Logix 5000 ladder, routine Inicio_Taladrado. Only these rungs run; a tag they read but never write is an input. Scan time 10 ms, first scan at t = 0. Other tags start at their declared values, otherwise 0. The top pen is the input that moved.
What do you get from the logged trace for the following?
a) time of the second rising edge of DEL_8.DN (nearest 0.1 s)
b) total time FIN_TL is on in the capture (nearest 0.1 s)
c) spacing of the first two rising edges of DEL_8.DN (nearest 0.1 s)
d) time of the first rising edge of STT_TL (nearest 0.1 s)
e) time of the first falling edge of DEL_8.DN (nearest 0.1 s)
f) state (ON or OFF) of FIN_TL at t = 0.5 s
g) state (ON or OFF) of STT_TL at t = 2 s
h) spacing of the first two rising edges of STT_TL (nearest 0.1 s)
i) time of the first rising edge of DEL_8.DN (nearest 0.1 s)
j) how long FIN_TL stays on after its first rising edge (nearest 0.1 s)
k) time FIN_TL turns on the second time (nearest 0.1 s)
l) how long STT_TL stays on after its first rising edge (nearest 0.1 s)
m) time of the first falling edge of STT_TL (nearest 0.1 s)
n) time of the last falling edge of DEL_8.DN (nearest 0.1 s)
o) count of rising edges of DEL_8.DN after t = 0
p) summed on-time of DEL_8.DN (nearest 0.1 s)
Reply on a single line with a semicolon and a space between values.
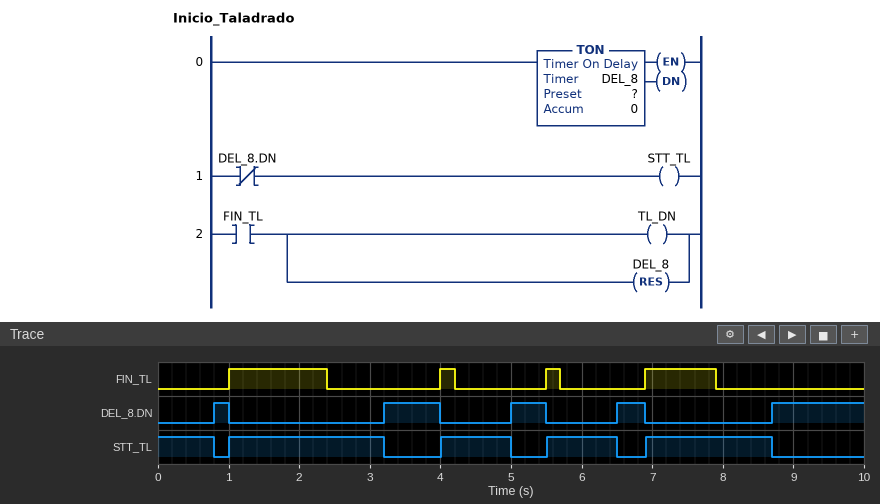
3.2 s; 2.8 s; 2.4 s; 1.0 s; 1.0 s; OFF; ON; 3.0 s; 0.8 s; 1.4 s; 4.0 s; 2.2 s; 0.8 s; 6.9 s; 5; 3.2 s
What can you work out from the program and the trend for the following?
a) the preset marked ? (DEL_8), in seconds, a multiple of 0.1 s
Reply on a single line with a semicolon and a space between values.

0.8 s
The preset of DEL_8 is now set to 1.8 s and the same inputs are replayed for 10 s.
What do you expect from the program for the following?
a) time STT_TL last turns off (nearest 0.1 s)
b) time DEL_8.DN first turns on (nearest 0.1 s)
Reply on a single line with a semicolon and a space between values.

9.7 s; 9.7 s
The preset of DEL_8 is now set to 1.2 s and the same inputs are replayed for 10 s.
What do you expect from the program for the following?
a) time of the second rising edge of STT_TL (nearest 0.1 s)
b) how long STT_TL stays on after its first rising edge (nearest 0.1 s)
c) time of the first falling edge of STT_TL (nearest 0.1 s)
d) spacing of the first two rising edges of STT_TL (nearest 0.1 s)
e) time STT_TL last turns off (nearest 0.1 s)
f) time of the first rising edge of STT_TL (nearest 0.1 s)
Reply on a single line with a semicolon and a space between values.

5.5 s; 1.4 s; 3.6 s; 1.5 s; 9.1 s; 4.0 s
